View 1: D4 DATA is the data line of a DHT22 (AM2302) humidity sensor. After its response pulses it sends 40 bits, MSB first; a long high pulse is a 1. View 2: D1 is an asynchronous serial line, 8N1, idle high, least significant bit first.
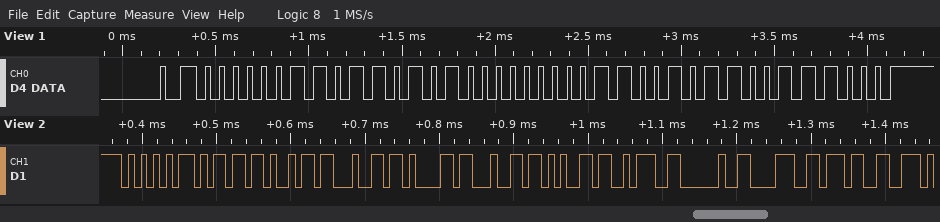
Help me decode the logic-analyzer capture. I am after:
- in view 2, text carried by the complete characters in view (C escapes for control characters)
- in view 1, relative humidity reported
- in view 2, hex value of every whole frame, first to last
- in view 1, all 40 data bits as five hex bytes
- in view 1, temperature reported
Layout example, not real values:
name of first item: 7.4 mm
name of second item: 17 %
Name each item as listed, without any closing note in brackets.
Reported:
in view 2, text carried by the complete characters in view: "Umidade: 87"
in view 1, relative humidity reported: 87.4 %
in view 2, hex value of every whole frame, first to last: 55 6D 69 64 61 64 65 3A 20 38 37
in view 1, all 40 data bits as five hex bytes: 03 6A 00 CB 38
in view 1, temperature reported: 20.3 °C
